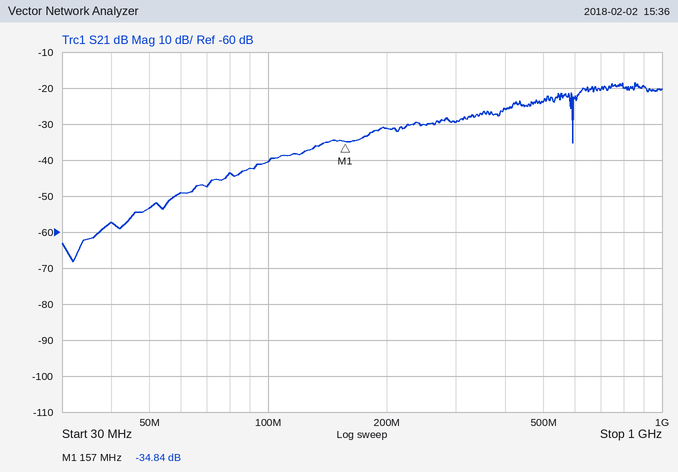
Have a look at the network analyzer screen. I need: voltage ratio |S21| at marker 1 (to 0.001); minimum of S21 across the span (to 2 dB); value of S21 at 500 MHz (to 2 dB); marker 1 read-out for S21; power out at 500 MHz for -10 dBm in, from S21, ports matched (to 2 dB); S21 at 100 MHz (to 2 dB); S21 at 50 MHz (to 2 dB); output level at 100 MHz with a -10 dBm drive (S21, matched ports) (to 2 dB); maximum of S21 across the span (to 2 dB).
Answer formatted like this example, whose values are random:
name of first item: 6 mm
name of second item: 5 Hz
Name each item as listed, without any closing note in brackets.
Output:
voltage ratio |S21| at marker 1: 0.018
minimum of S21 across the span: -68 dB
value of S21 at 500 MHz: -24 dB
marker 1 read-out for S21: -34.84 dB
power out at 500 MHz for -10 dBm in, from S21, ports matched: -34 dBm
S21 at 100 MHz: -40 dB
S21 at 50 MHz: -54 dB
output level at 100 MHz with a -10 dBm drive (S21, matched ports): -50 dBm
maximum of S21 across the span: -18 dB
